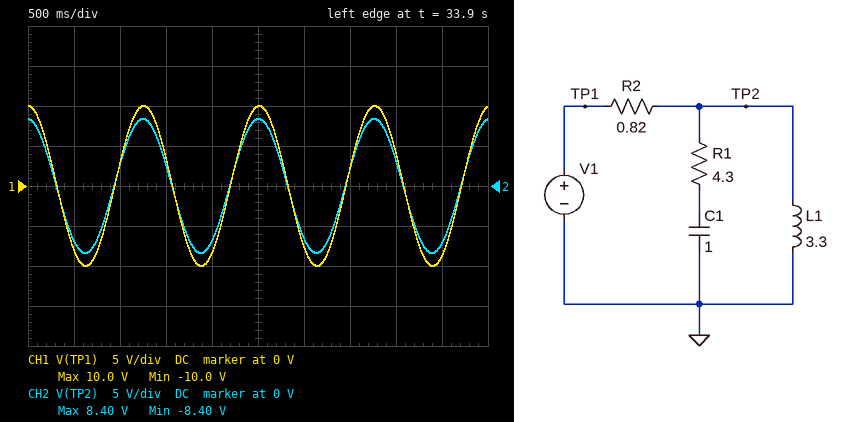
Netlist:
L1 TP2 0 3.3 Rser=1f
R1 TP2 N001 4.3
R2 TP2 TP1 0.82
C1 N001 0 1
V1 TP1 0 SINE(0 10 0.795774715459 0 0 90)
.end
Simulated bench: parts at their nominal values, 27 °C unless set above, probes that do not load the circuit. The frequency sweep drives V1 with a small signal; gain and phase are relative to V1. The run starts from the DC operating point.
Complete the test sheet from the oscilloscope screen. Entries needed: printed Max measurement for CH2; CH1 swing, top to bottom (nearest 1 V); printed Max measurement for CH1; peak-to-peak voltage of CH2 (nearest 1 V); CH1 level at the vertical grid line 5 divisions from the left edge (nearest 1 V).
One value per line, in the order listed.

8.40 V
20 V
10.0 V
17 V
10 V
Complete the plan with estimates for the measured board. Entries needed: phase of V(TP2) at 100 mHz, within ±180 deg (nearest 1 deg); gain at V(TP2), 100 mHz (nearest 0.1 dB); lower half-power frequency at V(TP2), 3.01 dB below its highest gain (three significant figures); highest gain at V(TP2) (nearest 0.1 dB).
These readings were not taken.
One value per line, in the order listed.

11 deg
-2.6 dB
30.8 mHz
-1.5 dB
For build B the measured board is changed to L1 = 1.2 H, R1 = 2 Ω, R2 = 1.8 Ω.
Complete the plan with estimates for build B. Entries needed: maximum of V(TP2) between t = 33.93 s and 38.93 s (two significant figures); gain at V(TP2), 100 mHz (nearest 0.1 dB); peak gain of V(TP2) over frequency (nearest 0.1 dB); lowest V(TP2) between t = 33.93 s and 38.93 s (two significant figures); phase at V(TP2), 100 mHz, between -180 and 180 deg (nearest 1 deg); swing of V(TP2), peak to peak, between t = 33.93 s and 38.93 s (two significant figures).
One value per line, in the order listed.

5.1 V
-8.7 dB
-5.6 dB
-5.1 V
9 deg
10 V
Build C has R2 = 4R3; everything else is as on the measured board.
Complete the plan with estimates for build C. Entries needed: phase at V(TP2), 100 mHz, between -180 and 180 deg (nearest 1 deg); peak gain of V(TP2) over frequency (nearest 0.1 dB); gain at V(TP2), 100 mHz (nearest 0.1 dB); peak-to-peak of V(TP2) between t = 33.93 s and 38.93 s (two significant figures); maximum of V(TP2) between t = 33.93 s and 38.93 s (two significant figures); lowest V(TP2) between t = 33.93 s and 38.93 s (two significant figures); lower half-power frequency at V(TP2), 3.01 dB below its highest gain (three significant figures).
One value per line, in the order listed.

27 deg
-6.0 dB
-9.6 dB
9.9 V
4.9 V
-4.9 V
116 mHz
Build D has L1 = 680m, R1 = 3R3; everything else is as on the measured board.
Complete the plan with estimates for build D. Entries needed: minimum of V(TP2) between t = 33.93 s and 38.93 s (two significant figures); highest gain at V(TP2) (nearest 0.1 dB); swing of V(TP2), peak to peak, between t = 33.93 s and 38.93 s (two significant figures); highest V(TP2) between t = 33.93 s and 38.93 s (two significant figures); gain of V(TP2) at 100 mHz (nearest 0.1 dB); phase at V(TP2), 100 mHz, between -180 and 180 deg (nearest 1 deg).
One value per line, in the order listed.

-7.5 V
-1.9 dB
15 V
7.5 V
-5.6 dB
6 deg
